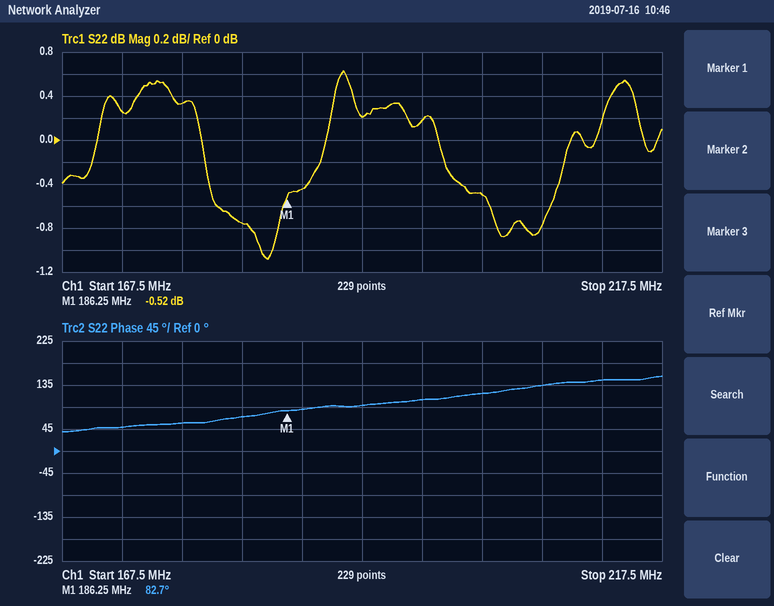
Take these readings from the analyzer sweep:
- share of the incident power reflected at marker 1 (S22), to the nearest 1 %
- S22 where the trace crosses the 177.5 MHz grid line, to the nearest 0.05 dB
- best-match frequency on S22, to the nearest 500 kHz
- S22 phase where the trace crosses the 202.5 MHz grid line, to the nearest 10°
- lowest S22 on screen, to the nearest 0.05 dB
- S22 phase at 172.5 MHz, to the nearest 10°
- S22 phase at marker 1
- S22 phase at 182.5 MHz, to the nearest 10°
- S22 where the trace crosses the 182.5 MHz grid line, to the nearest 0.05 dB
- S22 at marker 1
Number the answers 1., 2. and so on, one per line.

1. 89 %
2. 0.35 dB
3. 184.5 MHz
4. 120°
5. -1.10 dB
6. 50°
7. 82.7°
8. 70°
9. -0.75 dB
10. -0.52 dB
